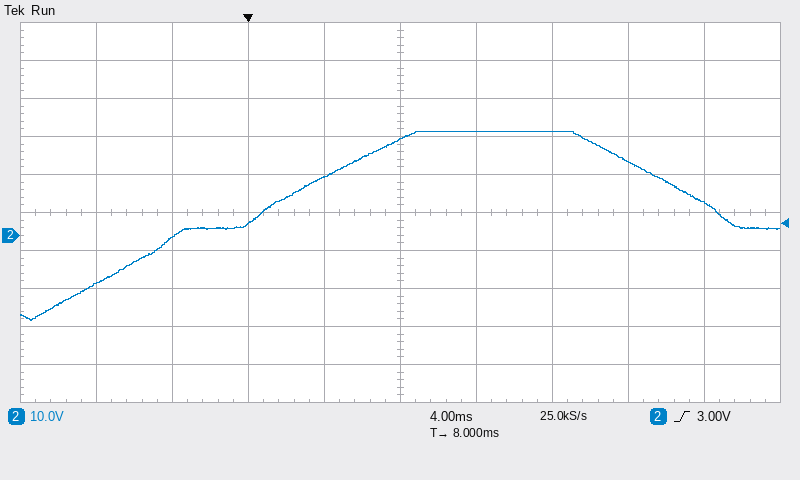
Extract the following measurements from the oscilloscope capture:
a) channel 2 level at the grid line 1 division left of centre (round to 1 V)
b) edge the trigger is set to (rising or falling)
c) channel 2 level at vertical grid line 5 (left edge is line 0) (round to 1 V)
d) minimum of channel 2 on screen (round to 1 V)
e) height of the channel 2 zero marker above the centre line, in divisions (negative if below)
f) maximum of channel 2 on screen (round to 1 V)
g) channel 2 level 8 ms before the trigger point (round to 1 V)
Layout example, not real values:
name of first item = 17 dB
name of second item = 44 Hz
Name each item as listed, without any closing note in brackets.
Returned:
channel 2 level at the grid line 1 division left of centre = 15 V
edge the trigger is set to = rising
channel 2 level at vertical grid line 5 (left edge is line 0) = 25 V
minimum of channel 2 on screen = -22 V
height of the channel 2 zero marker above the centre line, in divisions = -0.6 div
maximum of channel 2 on screen = 27 V
channel 2 level 8 ms before the trigger point = -13 V
